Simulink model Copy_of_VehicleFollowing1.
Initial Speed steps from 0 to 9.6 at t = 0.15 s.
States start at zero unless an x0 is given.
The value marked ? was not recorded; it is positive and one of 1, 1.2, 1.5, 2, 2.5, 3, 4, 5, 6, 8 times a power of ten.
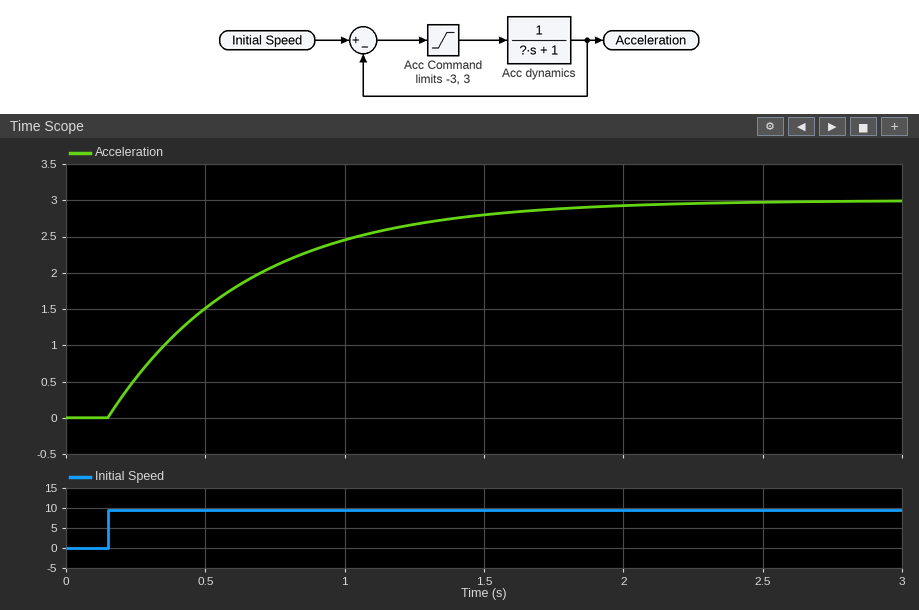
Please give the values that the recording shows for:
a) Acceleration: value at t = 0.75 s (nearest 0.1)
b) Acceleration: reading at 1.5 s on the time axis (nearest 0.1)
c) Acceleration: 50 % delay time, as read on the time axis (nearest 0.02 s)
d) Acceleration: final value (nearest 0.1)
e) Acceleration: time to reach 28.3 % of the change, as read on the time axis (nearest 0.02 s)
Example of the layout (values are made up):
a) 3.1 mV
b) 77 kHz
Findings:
a) 2.1
b) 2.8
c) 0.50 s
d) 3.0
e) 0.32 s
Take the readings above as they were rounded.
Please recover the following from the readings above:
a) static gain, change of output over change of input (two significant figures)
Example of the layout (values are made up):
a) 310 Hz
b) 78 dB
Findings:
a) 0.31
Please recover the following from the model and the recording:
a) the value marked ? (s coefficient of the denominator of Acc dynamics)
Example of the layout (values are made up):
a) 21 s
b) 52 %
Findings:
a) 0.5
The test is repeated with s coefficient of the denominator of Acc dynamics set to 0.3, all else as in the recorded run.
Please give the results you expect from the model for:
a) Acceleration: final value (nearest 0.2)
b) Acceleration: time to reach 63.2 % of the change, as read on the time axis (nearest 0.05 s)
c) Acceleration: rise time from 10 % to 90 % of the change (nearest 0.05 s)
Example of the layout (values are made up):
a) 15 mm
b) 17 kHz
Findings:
a) 3.0
b) 0.45 s
c) 0.65 s
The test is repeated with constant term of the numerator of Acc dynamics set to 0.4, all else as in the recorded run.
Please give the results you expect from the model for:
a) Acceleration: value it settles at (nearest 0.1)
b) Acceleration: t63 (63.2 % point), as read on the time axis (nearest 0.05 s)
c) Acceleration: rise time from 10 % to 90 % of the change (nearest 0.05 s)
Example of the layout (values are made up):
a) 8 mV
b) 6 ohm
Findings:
a) 1.2
b) 0.65 s
c) 1.10 s
